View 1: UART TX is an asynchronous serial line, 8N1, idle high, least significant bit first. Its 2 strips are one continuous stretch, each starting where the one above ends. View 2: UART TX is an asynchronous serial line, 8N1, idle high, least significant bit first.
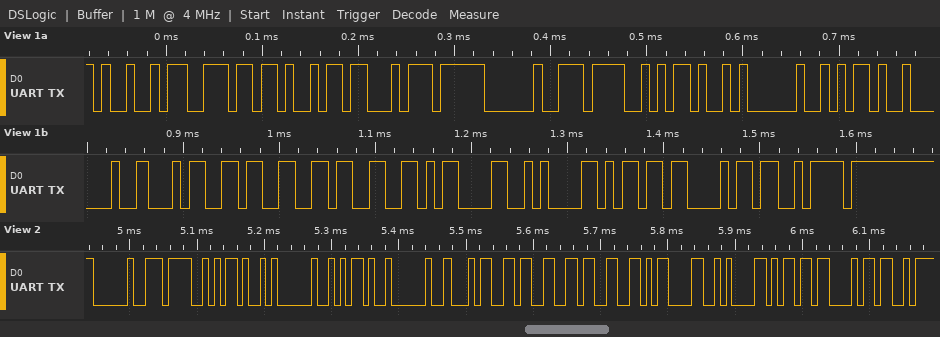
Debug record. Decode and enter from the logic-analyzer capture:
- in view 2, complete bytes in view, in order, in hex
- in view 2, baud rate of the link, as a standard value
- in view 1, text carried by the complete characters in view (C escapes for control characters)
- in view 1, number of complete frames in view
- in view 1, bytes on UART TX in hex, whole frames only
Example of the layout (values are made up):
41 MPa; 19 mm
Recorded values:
20 4F 4B 20 2D 20 34 33 33 0D 0A 6D 68; 115200 baud; "Init OK - 433\r\nmhz"; 18; 49 6E 69 74 20 4F 4B 20 2D 20 34 33 33 0D 0A 6D 68 7A
